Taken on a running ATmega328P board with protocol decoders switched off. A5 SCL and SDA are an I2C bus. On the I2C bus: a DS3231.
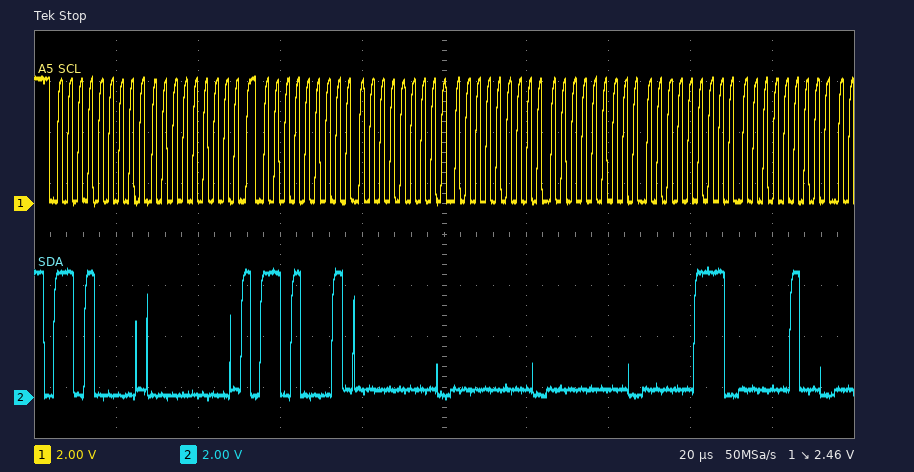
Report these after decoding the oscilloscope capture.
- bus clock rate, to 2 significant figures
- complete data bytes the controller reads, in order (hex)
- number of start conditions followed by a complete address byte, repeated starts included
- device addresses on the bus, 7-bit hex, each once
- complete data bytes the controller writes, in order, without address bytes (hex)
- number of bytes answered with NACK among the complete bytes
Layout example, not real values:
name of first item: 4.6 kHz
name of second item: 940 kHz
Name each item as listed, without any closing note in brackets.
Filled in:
bus clock rate, to 2 significant figures: 400 kHz
complete data bytes the controller reads, in order: 00 00 00 07 04
number of start conditions followed by a complete address byte, repeated starts included: 2
device addresses on the bus, 7-bit hex, each once: 0x68
complete data bytes the controller writes, in order, without address bytes: 00
number of bytes answered with NACK among the complete bytes: 0
